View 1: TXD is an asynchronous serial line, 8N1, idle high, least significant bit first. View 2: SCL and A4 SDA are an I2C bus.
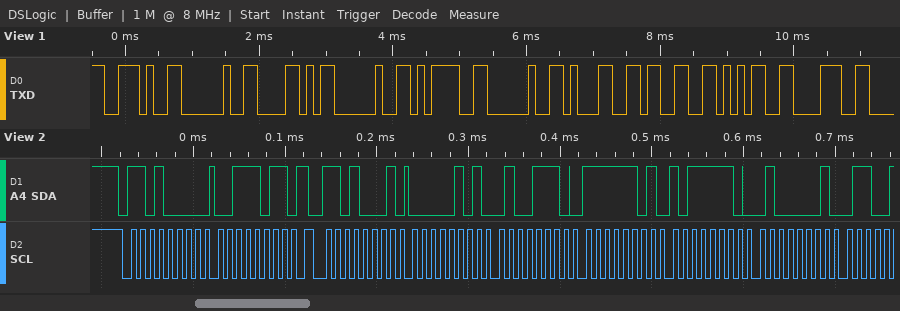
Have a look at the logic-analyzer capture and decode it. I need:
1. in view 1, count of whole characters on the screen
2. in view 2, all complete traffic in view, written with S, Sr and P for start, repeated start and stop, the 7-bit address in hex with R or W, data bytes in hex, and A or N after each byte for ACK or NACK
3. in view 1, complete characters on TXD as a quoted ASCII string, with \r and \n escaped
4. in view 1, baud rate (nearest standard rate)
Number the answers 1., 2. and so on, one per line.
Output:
1. 10
2. S 68W A 3B A Sr 68R A 05 A 4E A FD A BE A 41 A
3. ". X = 1358"
4. 9600 baud
